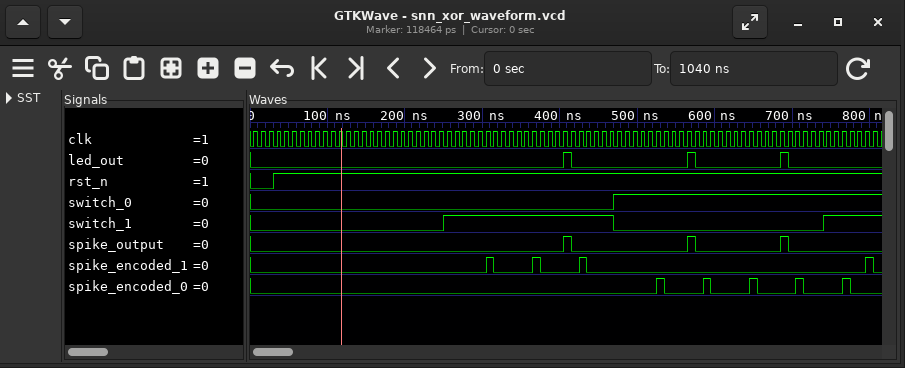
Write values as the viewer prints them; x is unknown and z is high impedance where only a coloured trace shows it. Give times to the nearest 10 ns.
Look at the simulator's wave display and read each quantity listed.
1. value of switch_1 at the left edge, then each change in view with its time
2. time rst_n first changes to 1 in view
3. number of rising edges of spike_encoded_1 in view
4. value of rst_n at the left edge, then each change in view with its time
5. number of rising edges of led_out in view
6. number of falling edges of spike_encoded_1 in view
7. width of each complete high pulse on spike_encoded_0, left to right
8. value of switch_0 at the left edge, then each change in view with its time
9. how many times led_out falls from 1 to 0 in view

0, 1 at 250 ns, 0 at 470 ns, 1 at 740 ns
30 ns
4
0, 1 at 30 ns
3
4
10 ns, 10 ns, 10 ns, 10 ns, 10 ns
0, 1 at 470 ns
3
